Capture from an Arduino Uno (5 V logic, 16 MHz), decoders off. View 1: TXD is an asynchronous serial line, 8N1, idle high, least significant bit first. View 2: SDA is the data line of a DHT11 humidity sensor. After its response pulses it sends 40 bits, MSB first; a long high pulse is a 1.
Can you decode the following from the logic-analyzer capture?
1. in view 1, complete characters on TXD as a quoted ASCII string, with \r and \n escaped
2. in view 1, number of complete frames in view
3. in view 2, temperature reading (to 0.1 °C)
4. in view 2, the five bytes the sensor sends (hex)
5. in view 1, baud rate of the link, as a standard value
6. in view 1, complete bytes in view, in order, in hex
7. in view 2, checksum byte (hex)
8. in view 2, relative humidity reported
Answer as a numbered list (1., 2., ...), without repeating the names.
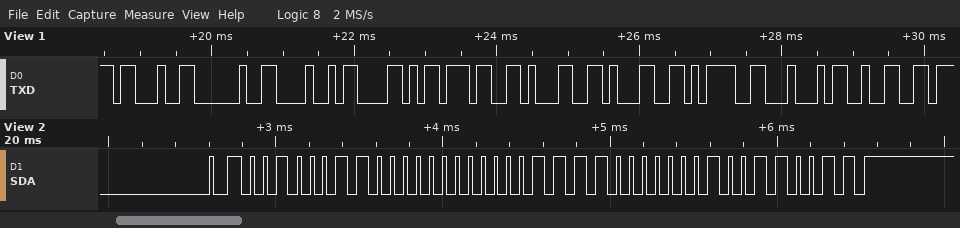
1. "# HX711=D2"
2. 10
3. 15.1 °C
4. 23 00 0F 01 33
5. 9600 baud
6. 23 20 48 58 37 31 31 3D 44 32
7. 0x33
8. 35 %
